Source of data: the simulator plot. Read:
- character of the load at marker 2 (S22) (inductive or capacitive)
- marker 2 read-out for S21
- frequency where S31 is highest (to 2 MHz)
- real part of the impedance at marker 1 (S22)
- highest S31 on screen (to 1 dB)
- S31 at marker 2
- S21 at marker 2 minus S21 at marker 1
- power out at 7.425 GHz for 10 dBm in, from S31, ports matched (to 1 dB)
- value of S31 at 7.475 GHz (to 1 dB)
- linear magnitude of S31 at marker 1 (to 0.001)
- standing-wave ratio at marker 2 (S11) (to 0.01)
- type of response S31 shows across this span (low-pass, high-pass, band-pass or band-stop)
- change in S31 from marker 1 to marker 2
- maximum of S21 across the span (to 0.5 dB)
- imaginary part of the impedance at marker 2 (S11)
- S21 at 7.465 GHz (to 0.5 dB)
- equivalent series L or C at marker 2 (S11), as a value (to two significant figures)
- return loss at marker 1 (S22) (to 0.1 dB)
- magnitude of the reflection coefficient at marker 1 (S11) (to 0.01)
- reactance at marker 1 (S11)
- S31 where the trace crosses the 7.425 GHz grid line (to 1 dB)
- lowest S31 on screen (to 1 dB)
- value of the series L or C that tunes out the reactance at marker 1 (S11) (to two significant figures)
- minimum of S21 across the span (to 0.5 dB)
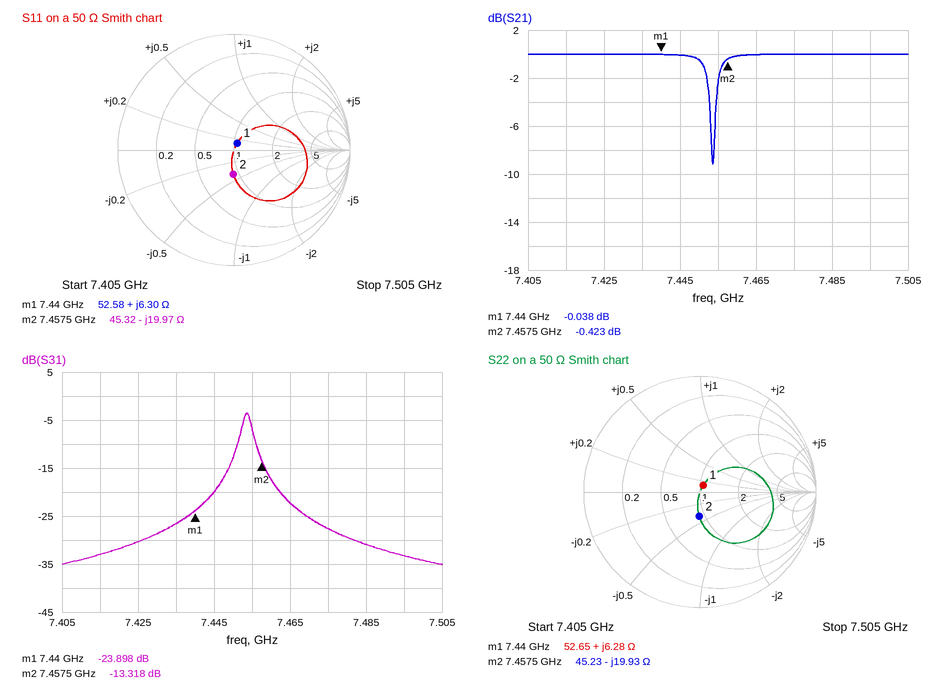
capacitive
-0.423 dB
7.454 GHz
52.65 Ω
-4 dB
-13.318 dB
-0.385 dB
-20 dBm
-28 dB
0.064
1.53
band-pass
10.580 dB
0.0 dB
-19.97 Ω
0.0 dB
1.1 pF
23.6 dB
0.07
+6.30 Ω
-30 dB
-35 dB
3.4 pF
-9.0 dB
